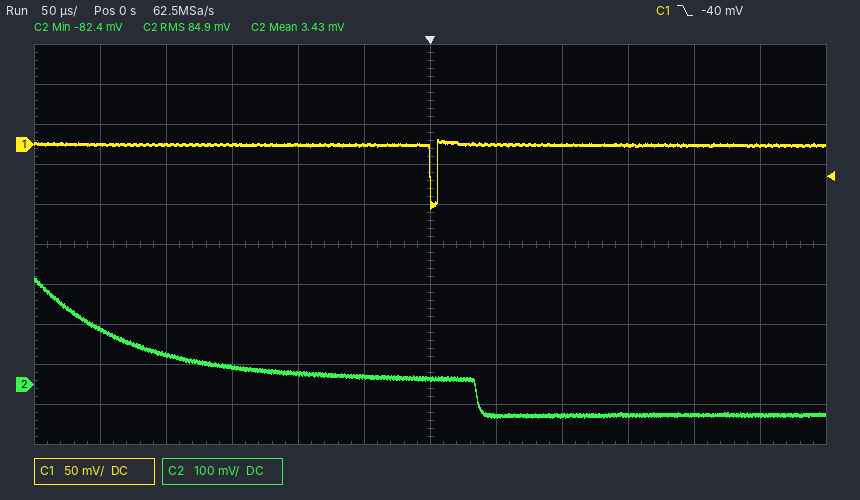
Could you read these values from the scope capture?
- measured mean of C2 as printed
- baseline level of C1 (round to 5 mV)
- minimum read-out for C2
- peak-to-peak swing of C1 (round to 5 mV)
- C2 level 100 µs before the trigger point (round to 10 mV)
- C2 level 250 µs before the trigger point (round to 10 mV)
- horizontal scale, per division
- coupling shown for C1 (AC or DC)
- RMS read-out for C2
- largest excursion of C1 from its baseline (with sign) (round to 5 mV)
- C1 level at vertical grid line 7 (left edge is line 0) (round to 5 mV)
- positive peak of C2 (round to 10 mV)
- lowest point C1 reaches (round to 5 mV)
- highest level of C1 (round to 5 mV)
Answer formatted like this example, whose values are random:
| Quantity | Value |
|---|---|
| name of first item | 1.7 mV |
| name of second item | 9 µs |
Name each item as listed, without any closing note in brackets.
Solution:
| Quantity | Value |
|---|---|
| measured mean of C2 as printed | 3.43 mV |
| baseline level of C1 | 0 mV |
| minimum read-out for C2 | -82.4 mV |
| peak-to-peak swing of C1 | 85 mV |
| C2 level 100 µs before the trigger point | 30 mV |
| C2 level 250 µs before the trigger point | 140 mV |
| horizontal scale, per division | 50 µs |
| coupling shown for C1 | DC |
| RMS read-out for C2 | 84.9 mV |
| largest excursion of C1 from its baseline (with sign) | -80 mV |
| C1 level at vertical grid line 7 (left edge is line 0) | 0 mV |
| positive peak of C2 | 270 mV |
| lowest point C1 reaches | -80 mV |
| highest level of C1 | 5 mV |
